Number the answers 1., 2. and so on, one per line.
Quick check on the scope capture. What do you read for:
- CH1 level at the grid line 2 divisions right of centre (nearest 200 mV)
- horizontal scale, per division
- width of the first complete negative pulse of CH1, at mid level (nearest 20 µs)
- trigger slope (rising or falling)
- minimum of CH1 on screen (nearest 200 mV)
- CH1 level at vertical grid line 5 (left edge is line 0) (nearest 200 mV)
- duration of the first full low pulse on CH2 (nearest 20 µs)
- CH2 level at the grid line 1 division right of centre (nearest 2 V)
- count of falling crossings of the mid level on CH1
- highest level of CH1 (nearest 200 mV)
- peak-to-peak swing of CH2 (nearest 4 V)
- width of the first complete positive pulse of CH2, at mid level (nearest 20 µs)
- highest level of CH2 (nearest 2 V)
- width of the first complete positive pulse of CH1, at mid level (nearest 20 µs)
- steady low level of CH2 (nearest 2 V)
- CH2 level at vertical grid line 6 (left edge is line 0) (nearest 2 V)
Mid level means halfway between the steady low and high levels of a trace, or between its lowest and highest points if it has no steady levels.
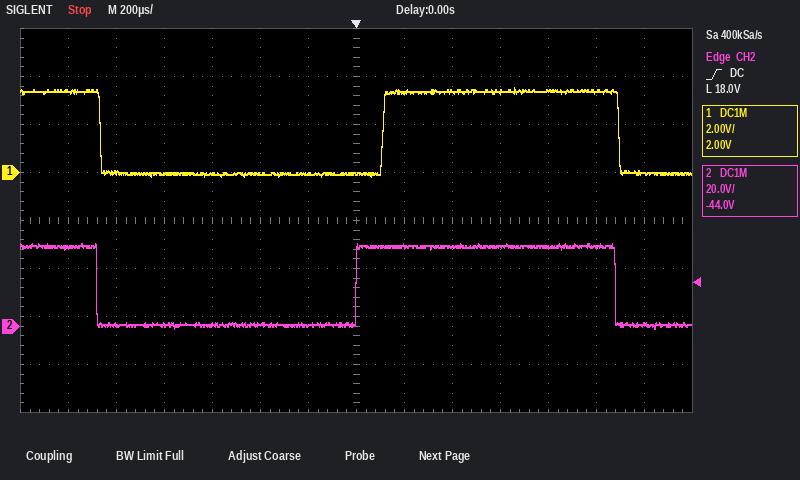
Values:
1. 3.4 V
2. 200 µs
3. 1.18 ms
4. rising
5. -200 mV
6. 0.0 V
7. 1.08 ms
8. 34 V
9. 2
10. 3.6 V
11. 36 V
12. 1.08 ms
13. 34 V
14. 980 µs
15. 0 V
16. 0 V
